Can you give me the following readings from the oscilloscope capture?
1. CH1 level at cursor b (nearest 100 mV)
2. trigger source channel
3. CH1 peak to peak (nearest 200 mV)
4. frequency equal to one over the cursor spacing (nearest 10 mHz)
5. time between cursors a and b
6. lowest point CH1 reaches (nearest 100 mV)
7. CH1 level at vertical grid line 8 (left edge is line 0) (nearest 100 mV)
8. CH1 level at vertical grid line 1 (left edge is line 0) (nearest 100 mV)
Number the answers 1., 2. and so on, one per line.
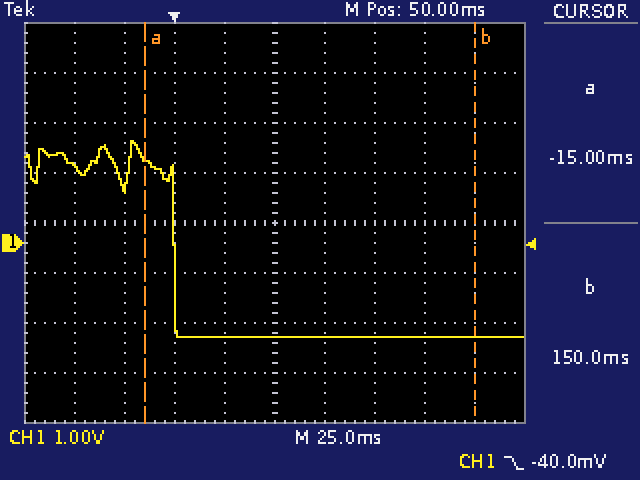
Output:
1. -1.9 V
2. CH1
3. 4.0 V
4. 6.06 Hz
5. 165.0 ms
6. -1.9 V
7. -1.9 V
8. 1.5 V
